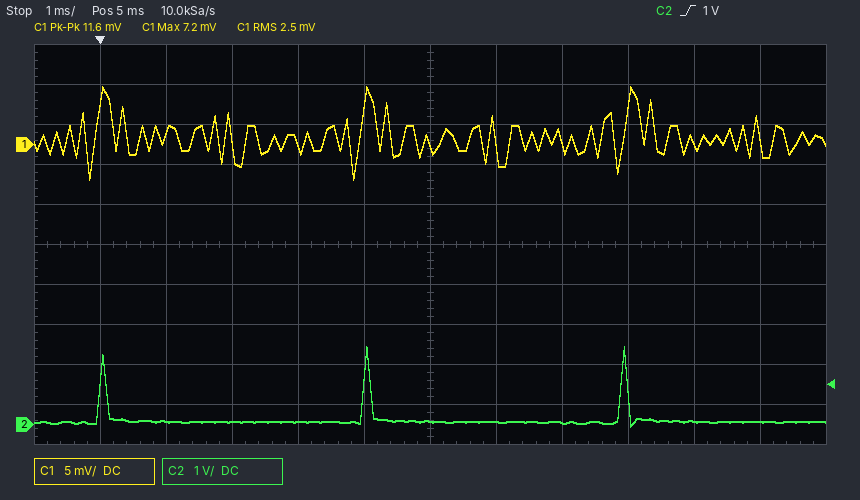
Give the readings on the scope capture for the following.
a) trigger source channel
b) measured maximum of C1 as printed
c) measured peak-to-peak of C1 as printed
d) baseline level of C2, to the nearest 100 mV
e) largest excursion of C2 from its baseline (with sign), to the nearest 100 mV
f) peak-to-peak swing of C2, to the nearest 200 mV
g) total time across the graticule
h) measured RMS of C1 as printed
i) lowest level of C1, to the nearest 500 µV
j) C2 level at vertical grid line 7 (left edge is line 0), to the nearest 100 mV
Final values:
C2
7.2 mV
11.6 mV
100 mV
+1.9 V
2.0 V
12 ms
2.5 mV
-4.5 mV
100 mV
